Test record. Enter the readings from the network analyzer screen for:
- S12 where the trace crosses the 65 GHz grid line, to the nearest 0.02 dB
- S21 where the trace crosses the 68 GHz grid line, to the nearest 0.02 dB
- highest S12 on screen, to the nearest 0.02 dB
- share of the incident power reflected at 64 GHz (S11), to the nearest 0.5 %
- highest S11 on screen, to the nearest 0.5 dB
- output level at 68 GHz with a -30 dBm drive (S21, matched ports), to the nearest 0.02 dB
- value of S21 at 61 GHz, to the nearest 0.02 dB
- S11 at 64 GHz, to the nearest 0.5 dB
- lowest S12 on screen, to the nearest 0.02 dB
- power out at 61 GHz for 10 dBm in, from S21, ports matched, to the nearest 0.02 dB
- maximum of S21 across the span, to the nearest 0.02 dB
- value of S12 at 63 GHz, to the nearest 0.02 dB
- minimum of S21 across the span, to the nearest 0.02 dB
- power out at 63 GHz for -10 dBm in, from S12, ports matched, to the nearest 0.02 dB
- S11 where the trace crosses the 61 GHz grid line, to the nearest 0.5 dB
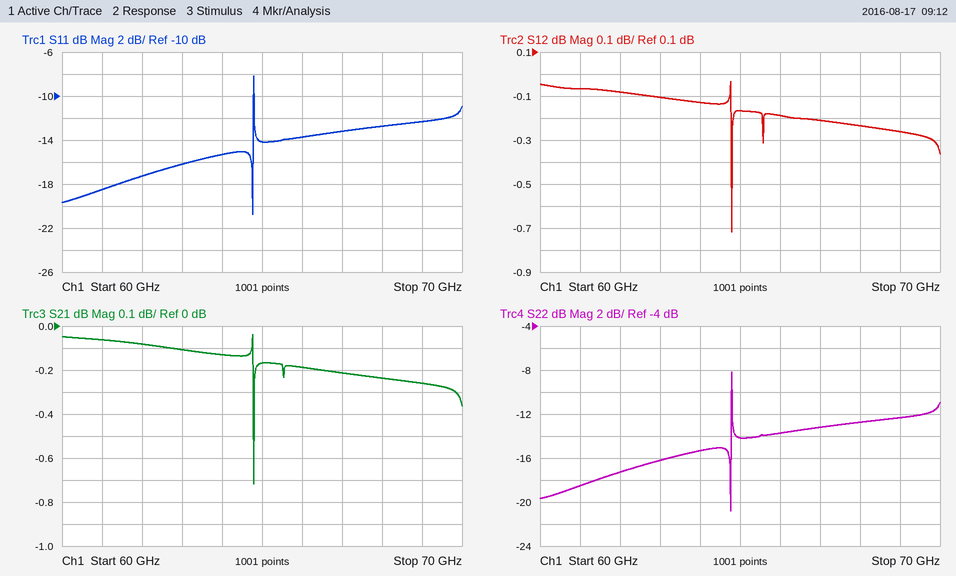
-0.16 dB
-0.24 dB
-0.04 dB
3.0 %
-8.0 dB
-30.24 dBm
-0.06 dB
-15.5 dB
-0.72 dB
9.94 dBm
-0.04 dB
-0.10 dB
-0.72 dB
-10.10 dBm
-18.5 dB
